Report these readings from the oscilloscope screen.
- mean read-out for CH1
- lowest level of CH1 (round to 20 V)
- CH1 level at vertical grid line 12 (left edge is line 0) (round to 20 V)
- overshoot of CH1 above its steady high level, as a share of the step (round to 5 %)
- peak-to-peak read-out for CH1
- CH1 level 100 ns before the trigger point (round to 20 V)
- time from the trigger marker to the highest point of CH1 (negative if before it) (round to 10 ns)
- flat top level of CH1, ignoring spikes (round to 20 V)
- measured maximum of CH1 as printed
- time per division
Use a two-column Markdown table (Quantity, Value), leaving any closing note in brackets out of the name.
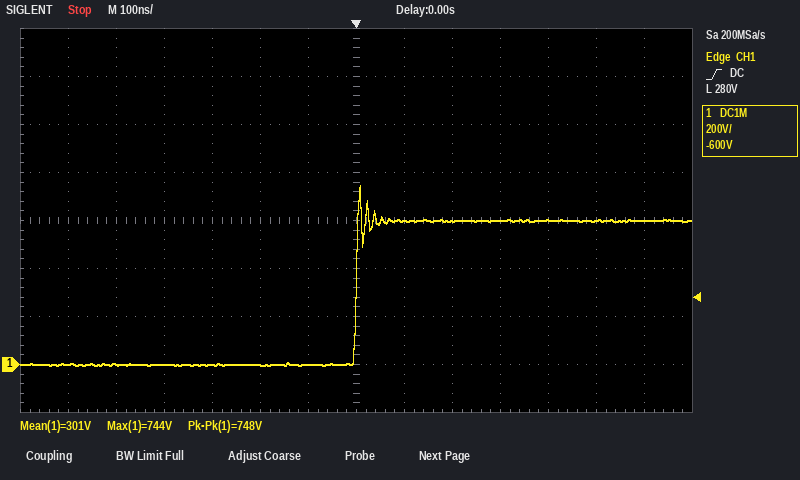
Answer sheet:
| Quantity | Value |
|---|---|
| mean read-out for CH1 | 301 V |
| lowest level of CH1 | 0 V |
| CH1 level at vertical grid line 12 (left edge is line 0) | 600 V |
| overshoot of CH1 above its steady high level, as a share of the step | 25 % |
| peak-to-peak read-out for CH1 | 748 V |
| CH1 level 100 ns before the trigger point | 0 V |
| time from the trigger marker to the highest point of CH1 (negative if before it) | +10 ns |
| flat top level of CH1, ignoring spikes | 600 V |
| measured maximum of CH1 as printed | 744 V |
| time per division | 100 ns |
